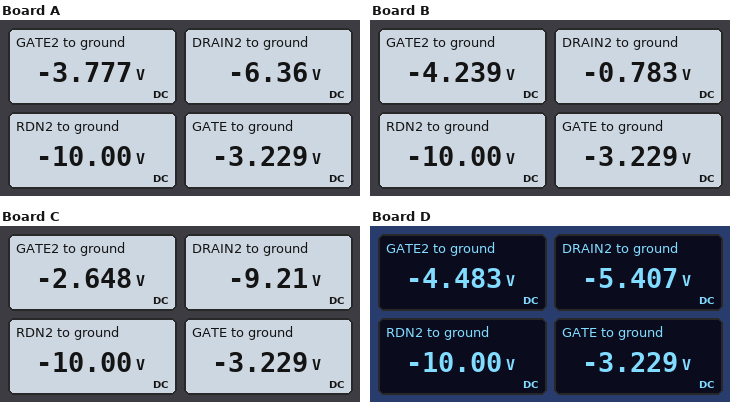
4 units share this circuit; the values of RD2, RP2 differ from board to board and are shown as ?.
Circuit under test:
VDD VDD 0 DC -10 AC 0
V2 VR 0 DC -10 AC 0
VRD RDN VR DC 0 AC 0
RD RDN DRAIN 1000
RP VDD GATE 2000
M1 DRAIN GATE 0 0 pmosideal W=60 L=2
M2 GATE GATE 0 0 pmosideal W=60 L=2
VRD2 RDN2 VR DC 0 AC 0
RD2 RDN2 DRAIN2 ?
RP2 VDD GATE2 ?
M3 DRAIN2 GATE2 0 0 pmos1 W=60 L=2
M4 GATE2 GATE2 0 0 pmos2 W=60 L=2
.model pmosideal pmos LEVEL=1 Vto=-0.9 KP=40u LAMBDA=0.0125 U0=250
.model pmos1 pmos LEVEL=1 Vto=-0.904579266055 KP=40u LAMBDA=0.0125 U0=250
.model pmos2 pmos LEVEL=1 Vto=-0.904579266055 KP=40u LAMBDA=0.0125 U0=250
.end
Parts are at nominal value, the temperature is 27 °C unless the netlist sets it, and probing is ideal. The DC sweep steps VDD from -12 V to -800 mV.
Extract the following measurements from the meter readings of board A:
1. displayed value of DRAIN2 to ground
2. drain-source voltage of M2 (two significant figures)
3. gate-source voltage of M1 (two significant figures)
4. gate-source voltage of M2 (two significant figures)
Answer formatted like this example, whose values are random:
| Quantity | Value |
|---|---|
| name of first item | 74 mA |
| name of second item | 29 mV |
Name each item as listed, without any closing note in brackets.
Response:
| Quantity | Value |
|---|---|
| displayed value of DRAIN2 to ground | -6.36 V |
| drain-source voltage of M2 | -3.2 V |
| gate-source voltage of M1 | -3.2 V |
| gate-source voltage of M2 | -3.2 V |
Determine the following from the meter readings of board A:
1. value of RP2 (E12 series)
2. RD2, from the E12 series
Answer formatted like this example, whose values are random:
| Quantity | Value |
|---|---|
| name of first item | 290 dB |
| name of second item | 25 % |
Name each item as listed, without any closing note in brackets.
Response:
| Quantity | Value |
|---|---|
| value of RP2 | 1.2 kΩ |
| RD2, from the E12 series | 680 Ω |
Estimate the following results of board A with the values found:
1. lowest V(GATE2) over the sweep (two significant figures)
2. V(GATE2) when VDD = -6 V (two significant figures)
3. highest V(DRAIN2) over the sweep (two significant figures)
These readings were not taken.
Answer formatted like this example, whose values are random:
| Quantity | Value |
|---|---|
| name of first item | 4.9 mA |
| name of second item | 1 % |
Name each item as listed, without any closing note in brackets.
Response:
| Quantity | Value |
|---|---|
| lowest V(GATE2) over the sweep | -4.1 V |
| V(GATE2) when VDD = -6 V | -2.9 V |
| highest V(DRAIN2) over the sweep | -5.5 V |
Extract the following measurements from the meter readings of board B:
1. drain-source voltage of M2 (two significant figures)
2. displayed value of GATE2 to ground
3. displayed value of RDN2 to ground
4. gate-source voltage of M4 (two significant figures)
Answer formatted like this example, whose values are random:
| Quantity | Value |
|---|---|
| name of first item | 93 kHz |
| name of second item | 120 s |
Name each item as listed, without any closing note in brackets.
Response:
| Quantity | Value |
|---|---|
| drain-source voltage of M2 | -3.2 V |
| displayed value of GATE2 to ground | -4.239 V |
| displayed value of RDN2 to ground | -10.00 V |
| gate-source voltage of M4 | -4.2 V |
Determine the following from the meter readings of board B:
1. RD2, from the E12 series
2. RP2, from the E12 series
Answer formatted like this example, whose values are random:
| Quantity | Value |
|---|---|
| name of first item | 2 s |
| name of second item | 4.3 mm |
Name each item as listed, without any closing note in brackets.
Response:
| Quantity | Value |
|---|---|
| RD2, from the E12 series | 3.3 kΩ |
| RP2, from the E12 series | 820 Ω |
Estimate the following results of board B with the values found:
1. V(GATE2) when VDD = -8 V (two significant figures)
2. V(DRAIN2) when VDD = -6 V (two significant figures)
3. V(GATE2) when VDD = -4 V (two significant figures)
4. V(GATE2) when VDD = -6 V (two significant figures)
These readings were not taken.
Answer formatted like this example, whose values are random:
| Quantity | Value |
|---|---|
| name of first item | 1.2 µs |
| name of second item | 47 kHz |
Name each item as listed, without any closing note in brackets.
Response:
| Quantity | Value |
|---|---|
| V(GATE2) when VDD = -8 V | -3.8 V |
| V(DRAIN2) when VDD = -6 V | -1.3 V |
| V(GATE2) when VDD = -4 V | -2.6 V |
| V(GATE2) when VDD = -6 V | -3.2 V |
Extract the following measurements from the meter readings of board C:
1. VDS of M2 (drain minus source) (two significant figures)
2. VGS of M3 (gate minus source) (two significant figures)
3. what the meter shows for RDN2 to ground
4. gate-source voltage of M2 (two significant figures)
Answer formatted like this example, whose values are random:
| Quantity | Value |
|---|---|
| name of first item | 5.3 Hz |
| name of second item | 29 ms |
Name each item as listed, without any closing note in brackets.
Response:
| Quantity | Value |
|---|---|
| VDS of M2 (drain minus source) | -3.2 V |
| VGS of M3 (gate minus source) | -2.6 V |
| what the meter shows for RDN2 to ground | -10.00 V |
| gate-source voltage of M2 | -3.2 V |
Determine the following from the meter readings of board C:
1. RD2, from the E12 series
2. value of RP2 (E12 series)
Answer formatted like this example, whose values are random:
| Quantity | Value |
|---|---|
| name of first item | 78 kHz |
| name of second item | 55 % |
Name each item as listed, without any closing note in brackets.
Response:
| Quantity | Value |
|---|---|
| RD2, from the E12 series | 390 Ω |
| value of RP2 | 3.9 kΩ |
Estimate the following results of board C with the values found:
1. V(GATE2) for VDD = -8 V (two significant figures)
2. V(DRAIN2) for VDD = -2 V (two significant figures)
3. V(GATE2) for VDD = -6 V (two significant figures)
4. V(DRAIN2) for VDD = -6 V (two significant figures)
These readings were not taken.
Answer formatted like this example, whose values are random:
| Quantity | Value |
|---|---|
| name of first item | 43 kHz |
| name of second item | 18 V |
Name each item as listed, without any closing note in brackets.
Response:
| Quantity | Value |
|---|---|
| V(GATE2) for VDD = -8 V | -2.4 V |
| V(DRAIN2) for VDD = -2 V | -9.9 V |
| V(GATE2) for VDD = -6 V | -2.2 V |
| V(DRAIN2) for VDD = -6 V | -9.6 V |
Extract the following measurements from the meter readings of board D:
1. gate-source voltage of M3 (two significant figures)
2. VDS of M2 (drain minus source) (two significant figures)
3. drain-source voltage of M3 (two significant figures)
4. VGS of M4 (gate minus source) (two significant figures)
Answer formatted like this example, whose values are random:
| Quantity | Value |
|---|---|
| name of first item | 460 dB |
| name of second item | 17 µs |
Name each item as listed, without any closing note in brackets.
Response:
| Quantity | Value |
|---|---|
| gate-source voltage of M3 | -4.5 V |
| VDS of M2 (drain minus source) | -3.2 V |
| drain-source voltage of M3 | -5.4 V |
| VGS of M4 (gate minus source) | -4.5 V |
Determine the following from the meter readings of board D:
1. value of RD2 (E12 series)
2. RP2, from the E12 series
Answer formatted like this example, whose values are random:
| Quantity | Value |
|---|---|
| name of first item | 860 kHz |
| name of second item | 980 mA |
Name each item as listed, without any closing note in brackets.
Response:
| Quantity | Value |
|---|---|
| value of RD2 | 560 Ω |
| RP2, from the E12 series | 680 Ω |
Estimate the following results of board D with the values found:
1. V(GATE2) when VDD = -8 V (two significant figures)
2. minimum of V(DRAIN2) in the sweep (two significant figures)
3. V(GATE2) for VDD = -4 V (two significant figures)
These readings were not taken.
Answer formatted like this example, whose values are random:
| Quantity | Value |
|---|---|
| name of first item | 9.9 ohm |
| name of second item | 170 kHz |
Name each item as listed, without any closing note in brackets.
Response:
| Quantity | Value |
|---|---|
| V(GATE2) when VDD = -8 V | -4.0 V |
| minimum of V(DRAIN2) in the sweep | -10 V |
| V(GATE2) for VDD = -4 V | -2.7 V |
